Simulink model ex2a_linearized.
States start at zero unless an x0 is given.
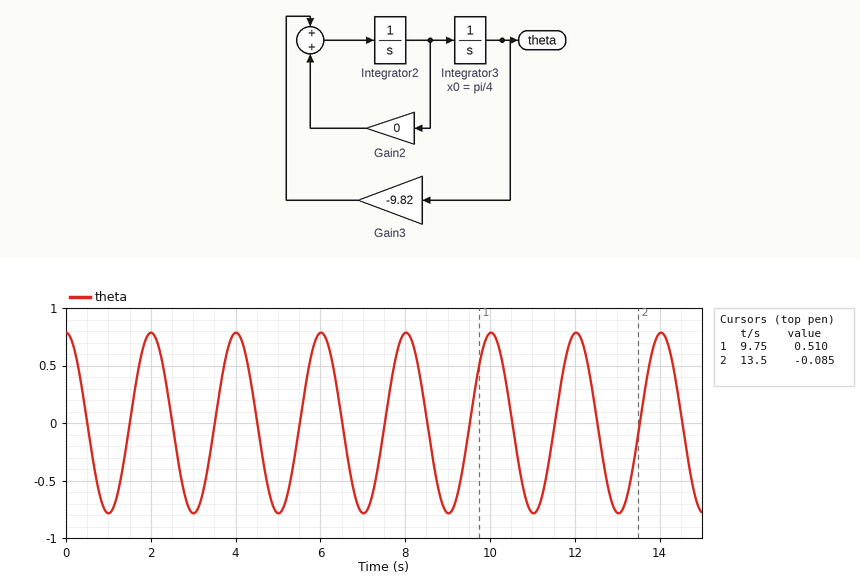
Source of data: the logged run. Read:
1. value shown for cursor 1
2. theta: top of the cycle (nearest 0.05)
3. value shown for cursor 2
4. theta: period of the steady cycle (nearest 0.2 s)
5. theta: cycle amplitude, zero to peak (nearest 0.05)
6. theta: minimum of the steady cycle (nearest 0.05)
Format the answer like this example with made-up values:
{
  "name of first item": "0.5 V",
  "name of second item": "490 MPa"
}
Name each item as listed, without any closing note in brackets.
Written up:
{
  "value shown for cursor 1": "0.510",
  "theta: top of the cycle": "0.80",
  "value shown for cursor 2": "-0.085",
  "theta: period of the steady cycle": "2.0 s",
  "theta: cycle amplitude, zero to peak": "0.80",
  "theta: minimum of the steady cycle": "-0.80"
}
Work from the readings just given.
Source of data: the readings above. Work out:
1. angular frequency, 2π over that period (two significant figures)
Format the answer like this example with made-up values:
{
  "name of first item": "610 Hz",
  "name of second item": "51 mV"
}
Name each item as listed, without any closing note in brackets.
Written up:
{
  "angular frequency, 2π over that period": "3.1 rad/s"
}
